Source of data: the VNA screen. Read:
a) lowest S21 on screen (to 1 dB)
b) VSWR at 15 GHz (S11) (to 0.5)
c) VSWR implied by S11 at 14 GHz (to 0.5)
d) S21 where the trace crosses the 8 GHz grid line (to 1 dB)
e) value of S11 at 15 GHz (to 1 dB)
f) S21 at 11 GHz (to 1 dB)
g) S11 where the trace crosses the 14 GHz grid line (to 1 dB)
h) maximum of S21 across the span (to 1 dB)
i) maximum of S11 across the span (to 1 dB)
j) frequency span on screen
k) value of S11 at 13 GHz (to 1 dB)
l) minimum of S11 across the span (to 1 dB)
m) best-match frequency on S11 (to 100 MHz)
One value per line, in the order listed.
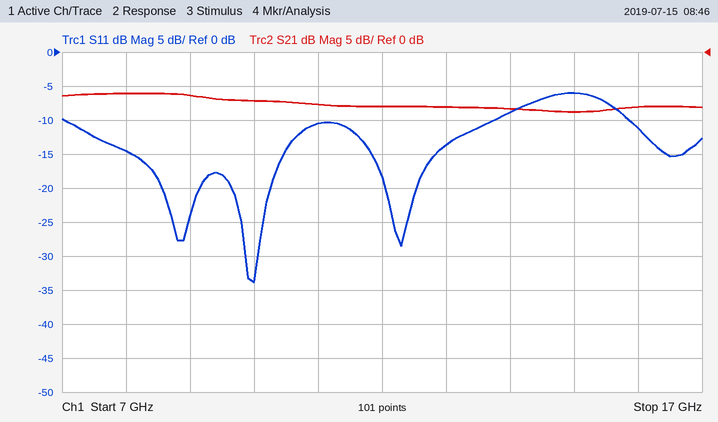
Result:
-9 dB
3.0
2.0
-6 dB
-6 dB
-8 dB
-9 dB
-6 dB
-6 dB
10 GHz
-14 dB
-34 dB
10.0 GHz
